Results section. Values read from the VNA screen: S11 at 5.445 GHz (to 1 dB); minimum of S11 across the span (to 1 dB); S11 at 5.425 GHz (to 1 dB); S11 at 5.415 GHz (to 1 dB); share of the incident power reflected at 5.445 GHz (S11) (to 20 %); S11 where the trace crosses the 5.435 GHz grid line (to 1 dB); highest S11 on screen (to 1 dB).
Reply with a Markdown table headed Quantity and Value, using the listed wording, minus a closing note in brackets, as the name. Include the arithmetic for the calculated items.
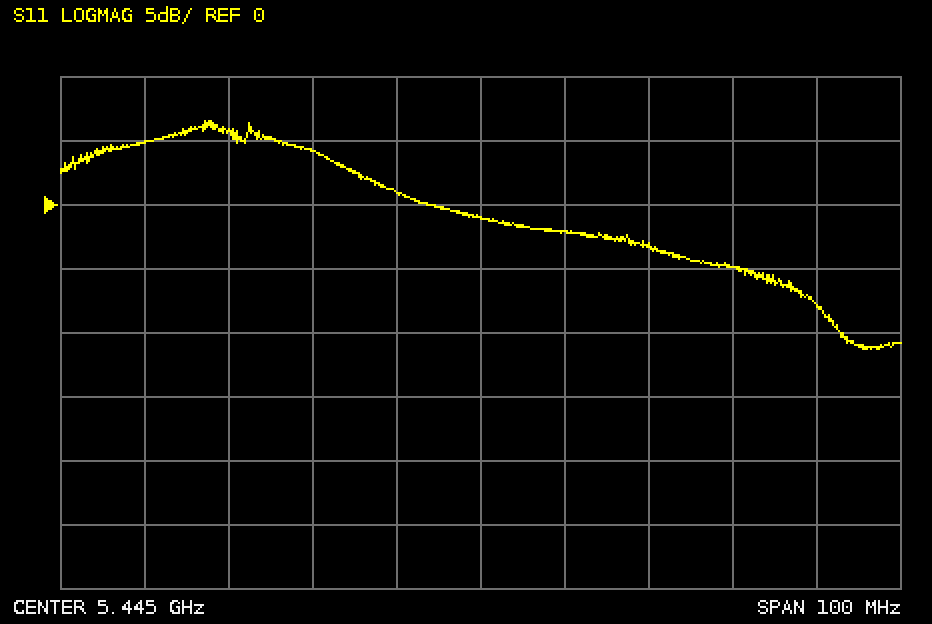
| Quantity | Value |
|---|---|
| S11 at 5.445 GHz | -1 dB |
| minimum of S11 across the span | -11 dB |
| S11 at 5.425 GHz | 4 dB |
| S11 at 5.415 GHz | 6 dB |
| share of the incident power reflected at 5.445 GHz (S11) | 10^(-1/10) ≈ 79.4 %, so 80 % to the nearest 20 % |
| S11 where the trace crosses the 5.435 GHz grid line | 1 dB |
| highest S11 on screen | 7 dB |
